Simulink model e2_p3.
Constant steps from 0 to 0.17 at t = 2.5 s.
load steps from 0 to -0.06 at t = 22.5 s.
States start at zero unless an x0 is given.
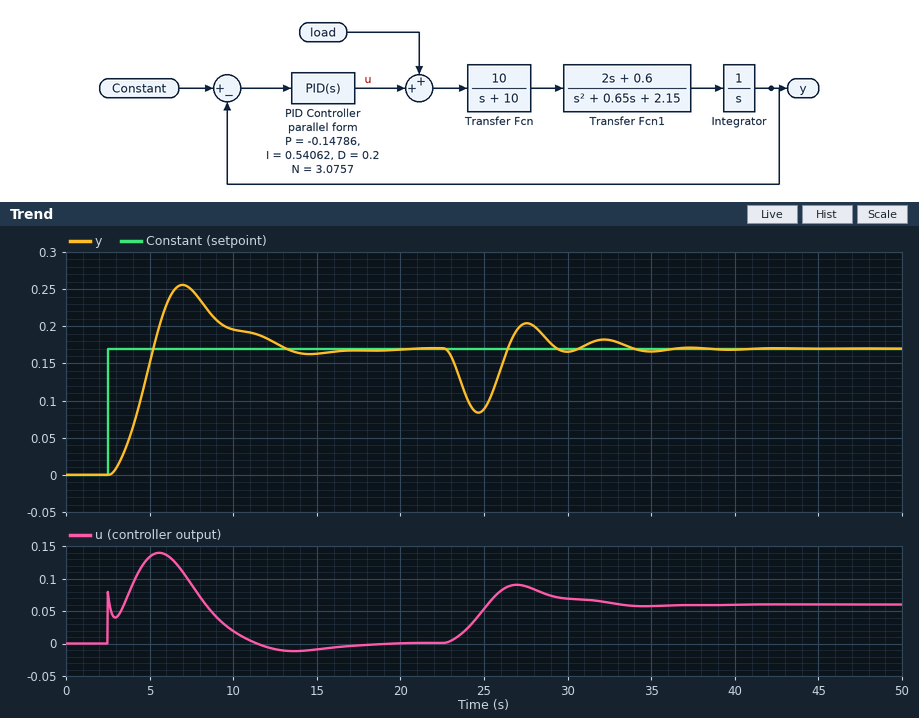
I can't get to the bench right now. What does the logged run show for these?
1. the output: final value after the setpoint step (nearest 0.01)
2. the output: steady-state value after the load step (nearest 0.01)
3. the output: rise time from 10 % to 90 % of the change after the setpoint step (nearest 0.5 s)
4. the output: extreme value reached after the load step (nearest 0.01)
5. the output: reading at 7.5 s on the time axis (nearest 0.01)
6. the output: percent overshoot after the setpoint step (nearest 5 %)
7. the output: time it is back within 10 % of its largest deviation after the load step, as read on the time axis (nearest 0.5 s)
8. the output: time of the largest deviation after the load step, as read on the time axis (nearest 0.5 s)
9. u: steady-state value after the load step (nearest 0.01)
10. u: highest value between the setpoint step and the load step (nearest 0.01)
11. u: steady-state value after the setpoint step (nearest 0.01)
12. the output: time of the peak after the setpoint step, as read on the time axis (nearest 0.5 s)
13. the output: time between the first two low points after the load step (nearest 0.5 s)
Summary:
0.17
0.17
2.0 s
0.08
0.25
50 %
33.0 s
24.5 s
0.06
0.14
0.00
7.0 s
5.5 s
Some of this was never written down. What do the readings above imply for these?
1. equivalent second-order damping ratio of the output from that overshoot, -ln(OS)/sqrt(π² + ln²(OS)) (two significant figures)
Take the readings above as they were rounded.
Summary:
0.22
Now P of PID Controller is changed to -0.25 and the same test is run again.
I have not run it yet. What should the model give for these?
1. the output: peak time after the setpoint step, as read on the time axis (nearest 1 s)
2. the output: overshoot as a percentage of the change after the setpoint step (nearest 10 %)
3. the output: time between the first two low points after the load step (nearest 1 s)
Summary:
7 s
70 %
6 s
